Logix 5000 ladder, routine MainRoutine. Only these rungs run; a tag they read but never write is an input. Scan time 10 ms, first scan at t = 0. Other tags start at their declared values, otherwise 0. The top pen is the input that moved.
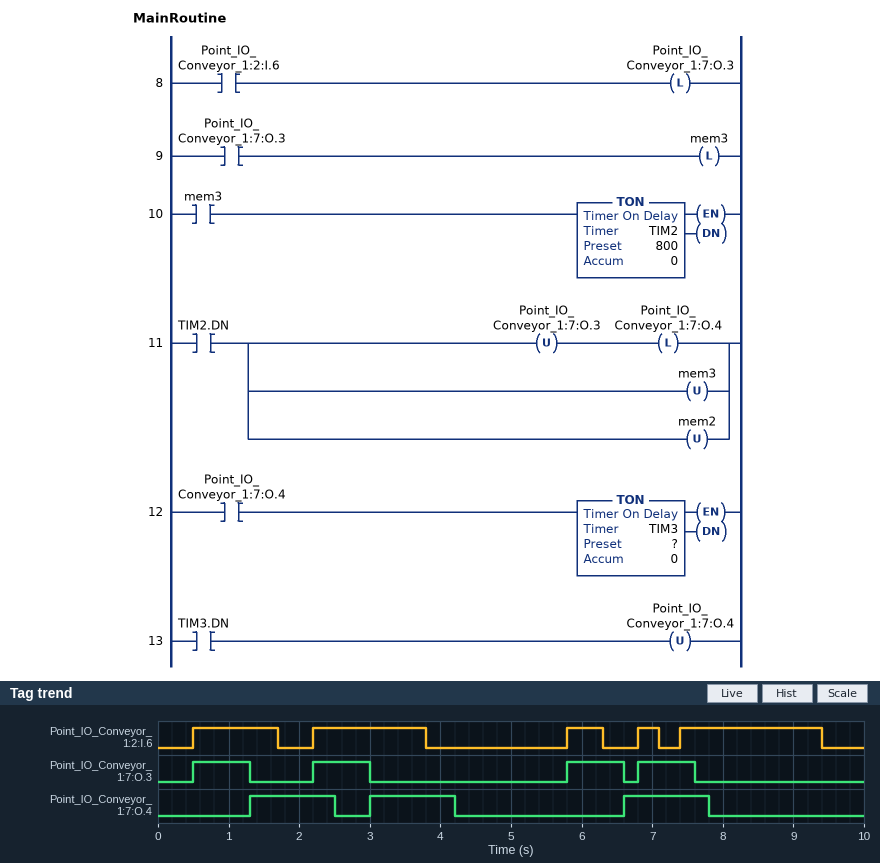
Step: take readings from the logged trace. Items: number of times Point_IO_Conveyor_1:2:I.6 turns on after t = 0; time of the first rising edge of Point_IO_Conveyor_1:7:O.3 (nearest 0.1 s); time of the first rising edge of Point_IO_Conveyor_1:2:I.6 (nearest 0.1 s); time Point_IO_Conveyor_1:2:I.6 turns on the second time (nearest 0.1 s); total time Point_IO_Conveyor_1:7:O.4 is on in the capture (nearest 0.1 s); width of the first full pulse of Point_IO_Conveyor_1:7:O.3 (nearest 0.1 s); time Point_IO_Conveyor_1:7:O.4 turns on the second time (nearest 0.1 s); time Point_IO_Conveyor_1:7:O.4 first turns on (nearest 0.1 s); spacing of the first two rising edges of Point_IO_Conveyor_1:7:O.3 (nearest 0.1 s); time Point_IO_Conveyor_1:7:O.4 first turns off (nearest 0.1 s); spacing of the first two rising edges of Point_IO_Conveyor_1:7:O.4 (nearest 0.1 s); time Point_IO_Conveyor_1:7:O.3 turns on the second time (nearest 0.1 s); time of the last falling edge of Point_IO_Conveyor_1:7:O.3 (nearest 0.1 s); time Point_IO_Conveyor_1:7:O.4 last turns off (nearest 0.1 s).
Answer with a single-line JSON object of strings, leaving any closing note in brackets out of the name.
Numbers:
{"number of times Point_IO_Conveyor_1:2:I.6 turns on after t = 0": "5", "time of the first rising edge of Point_IO_Conveyor_1:7:O.3": "0.5 s", "time of the first rising edge of Point_IO_Conveyor_1:2:I.6": "0.5 s", "time Point_IO_Conveyor_1:2:I.6 turns on the second time": "2.2 s", "total time Point_IO_Conveyor_1:7:O.4 is on in the capture": "3.6 s", "width of the first full pulse of Point_IO_Conveyor_1:7:O.3": "0.8 s", "time Point_IO_Conveyor_1:7:O.4 turns on the second time": "3.0 s", "time Point_IO_Conveyor_1:7:O.4 first turns on": "1.3 s", "spacing of the first two rising edges of Point_IO_Conveyor_1:7:O.3": "1.7 s", "time Point_IO_Conveyor_1:7:O.4 first turns off": "2.5 s", "spacing of the first two rising edges of Point_IO_Conveyor_1:7:O.4": "1.7 s", "time Point_IO_Conveyor_1:7:O.3 turns on the second time": "2.2 s", "time of the last falling edge of Point_IO_Conveyor_1:7:O.3": "7.6 s", "time Point_IO_Conveyor_1:7:O.4 last turns off": "7.8 s"}
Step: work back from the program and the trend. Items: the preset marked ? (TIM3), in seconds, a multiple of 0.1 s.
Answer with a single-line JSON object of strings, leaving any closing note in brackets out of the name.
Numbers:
{"the preset marked ? (TIM3), in seconds, a multiple of 0.1 s": "1.2 s"}
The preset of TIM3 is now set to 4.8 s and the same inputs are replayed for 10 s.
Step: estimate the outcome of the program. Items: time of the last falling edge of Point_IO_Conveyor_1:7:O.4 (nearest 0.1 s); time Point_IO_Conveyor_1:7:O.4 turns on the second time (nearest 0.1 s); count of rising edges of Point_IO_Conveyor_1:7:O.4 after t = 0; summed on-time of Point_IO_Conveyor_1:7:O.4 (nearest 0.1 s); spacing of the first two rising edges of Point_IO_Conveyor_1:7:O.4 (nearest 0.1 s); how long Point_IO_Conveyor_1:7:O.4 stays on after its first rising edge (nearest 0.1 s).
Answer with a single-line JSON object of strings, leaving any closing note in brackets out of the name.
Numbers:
{"time of the last falling edge of Point_IO_Conveyor_1:7:O.4": "6.1 s", "time Point_IO_Conveyor_1:7:O.4 turns on the second time": "6.6 s", "count of rising edges of Point_IO_Conveyor_1:7:O.4 after t = 0": "2", "summed on-time of Point_IO_Conveyor_1:7:O.4": "8.2 s", "spacing of the first two rising edges of Point_IO_Conveyor_1:7:O.4": "5.3 s", "how long Point_IO_Conveyor_1:7:O.4 stays on after its first rising edge": "4.8 s"}
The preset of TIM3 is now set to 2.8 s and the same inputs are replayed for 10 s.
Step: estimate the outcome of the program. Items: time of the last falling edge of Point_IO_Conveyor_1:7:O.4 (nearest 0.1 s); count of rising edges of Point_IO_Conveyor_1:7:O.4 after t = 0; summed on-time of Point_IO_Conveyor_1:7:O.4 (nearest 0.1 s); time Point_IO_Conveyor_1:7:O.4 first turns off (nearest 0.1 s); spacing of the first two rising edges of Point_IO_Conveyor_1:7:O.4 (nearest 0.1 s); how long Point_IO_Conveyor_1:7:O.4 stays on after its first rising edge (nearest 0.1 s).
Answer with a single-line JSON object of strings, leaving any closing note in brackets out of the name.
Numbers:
{"time of the last falling edge of Point_IO_Conveyor_1:7:O.4": "9.4 s", "count of rising edges of Point_IO_Conveyor_1:7:O.4 after t = 0": "2", "summed on-time of Point_IO_Conveyor_1:7:O.4": "5.6 s", "time Point_IO_Conveyor_1:7:O.4 first turns off": "4.1 s", "spacing of the first two rising edges of Point_IO_Conveyor_1:7:O.4": "5.3 s", "how long Point_IO_Conveyor_1:7:O.4 stays on after its first rising edge": "2.8 s"}
